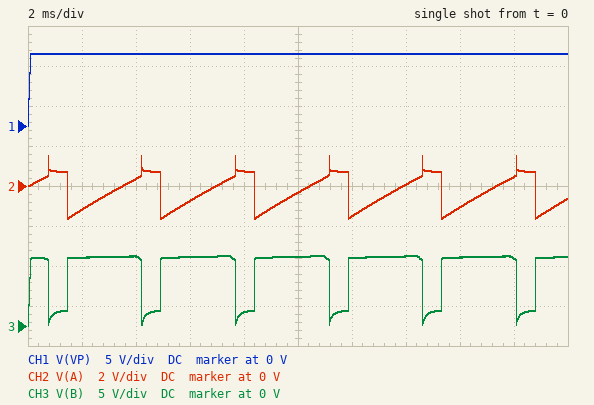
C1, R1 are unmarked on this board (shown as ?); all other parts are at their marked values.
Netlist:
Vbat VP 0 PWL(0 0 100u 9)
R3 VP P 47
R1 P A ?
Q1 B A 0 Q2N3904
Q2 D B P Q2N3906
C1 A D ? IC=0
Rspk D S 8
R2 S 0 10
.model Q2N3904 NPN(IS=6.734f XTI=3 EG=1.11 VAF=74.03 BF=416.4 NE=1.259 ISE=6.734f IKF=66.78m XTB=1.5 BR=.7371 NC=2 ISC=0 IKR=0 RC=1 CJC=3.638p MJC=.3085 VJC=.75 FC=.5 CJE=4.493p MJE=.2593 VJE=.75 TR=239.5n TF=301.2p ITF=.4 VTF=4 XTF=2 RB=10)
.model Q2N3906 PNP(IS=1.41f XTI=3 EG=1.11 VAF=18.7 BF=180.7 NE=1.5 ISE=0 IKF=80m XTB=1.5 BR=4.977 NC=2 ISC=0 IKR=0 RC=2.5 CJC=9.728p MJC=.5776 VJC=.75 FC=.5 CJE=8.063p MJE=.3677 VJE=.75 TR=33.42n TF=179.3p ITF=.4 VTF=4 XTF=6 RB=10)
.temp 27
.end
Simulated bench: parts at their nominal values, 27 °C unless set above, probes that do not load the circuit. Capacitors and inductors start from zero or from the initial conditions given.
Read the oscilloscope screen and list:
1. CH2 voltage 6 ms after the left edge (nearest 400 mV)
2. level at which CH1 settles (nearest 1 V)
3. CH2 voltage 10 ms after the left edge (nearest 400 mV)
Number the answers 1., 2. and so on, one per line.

1. -800 mV
2. 9 V
3. -400 mV
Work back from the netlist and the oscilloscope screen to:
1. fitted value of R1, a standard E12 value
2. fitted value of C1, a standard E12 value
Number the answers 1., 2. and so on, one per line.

1. 180 kΩ
2. 68 nF
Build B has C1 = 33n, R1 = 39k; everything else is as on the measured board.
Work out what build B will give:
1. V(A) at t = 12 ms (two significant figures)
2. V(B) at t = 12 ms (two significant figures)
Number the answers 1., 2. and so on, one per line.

1. 720 mV
2. 1.7 V
